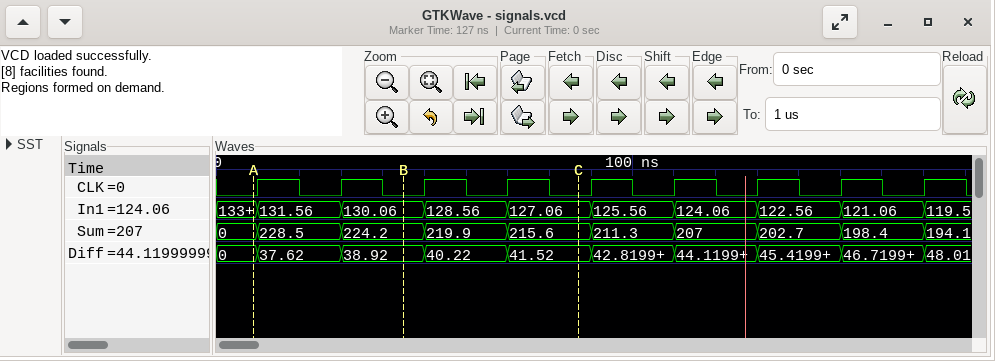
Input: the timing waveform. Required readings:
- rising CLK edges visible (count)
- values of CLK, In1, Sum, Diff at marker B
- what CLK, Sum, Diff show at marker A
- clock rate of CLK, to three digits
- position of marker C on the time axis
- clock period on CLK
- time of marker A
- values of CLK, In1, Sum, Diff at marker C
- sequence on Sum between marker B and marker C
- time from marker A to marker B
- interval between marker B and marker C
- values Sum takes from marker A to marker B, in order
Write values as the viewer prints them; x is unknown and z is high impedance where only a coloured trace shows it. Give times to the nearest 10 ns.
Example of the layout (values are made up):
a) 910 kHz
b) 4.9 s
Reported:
a) 9
b) CLK=0, In1=130.06, Sum=224.2, Diff=38.92
c) CLK=0, Sum=0, Diff=0
d) 50.0 MHz
e) 90 ns
f) 20 ns
g) 10 ns
h) CLK=0, In1=127.06, Sum=215.6, Diff=41.52
i) 224.2, 219.9, 215.6
j) 40 ns
k) 40 ns
l) 0, 228.5, 224.2
